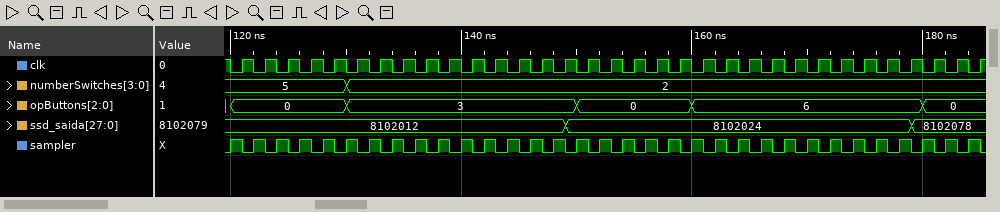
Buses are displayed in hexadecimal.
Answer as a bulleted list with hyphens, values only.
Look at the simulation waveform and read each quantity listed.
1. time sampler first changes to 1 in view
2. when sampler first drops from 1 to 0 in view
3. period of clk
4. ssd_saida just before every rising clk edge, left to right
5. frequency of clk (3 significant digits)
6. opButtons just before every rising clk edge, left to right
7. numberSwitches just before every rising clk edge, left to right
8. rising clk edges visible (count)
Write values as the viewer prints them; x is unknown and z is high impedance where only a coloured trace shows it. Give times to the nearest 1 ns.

- 120 ns
- 121 ns
- 2 ns
- 8102012, 8102012, 8102012, 8102012, 8102012, 8102012, 8102012, 8102012, 8102012, 8102012, 8102012, 8102012, 8102012, 8102012, 8102012, 8102024, 8102024, 8102024, 8102024, 8102024, 8102024, 8102024, 8102024, 8102024, 8102024, 8102024, 8102024, 8102024, 8102024, 8102024, 8102078, 8102078, 8102078
- 500 MHz
- 0, 0, 0, 0, 0, 3, 3, 3, 3, 3, 3, 3, 3, 3, 3, 0, 0, 0, 0, 0, 6, 6, 6, 6, 6, 6, 6, 6, 6, 6, 0, 0, 0
- 5, 5, 5, 5, 5, 2, 2, 2, 2, 2, 2, 2, 2, 2, 2, 2, 2, 2, 2, 2, 2, 2, 2, 2, 2, 2, 2, 2, 2, 2, 2, 2, 2
- 33
